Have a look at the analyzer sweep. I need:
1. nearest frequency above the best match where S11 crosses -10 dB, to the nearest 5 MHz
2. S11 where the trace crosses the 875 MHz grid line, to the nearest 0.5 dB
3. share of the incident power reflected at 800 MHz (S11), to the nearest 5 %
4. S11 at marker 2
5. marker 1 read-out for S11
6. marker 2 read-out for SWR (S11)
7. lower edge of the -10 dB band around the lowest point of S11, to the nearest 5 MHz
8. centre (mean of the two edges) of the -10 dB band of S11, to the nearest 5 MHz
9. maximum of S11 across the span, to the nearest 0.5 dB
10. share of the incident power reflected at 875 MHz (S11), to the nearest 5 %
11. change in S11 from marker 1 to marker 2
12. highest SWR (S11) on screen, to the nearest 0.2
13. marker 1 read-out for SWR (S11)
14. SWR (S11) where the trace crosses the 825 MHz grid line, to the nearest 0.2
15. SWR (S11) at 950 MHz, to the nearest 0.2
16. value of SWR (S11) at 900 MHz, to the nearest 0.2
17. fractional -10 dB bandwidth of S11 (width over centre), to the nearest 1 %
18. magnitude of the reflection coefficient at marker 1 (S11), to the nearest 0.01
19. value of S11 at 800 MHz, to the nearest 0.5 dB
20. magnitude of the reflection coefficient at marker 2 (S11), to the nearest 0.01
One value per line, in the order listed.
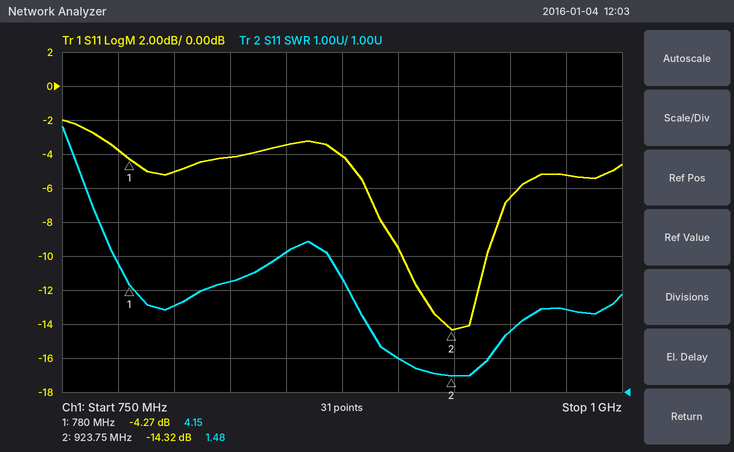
940 MHz
-4.0 dB
30 %
-14.32 dB
-4.27 dB
1.48
900 MHz
920 MHz
-2.0 dB
40 %
-10.05 dB
8.8
4.15
4.2
2.8
2.0
4 %
0.61
-5.0 dB
0.19
